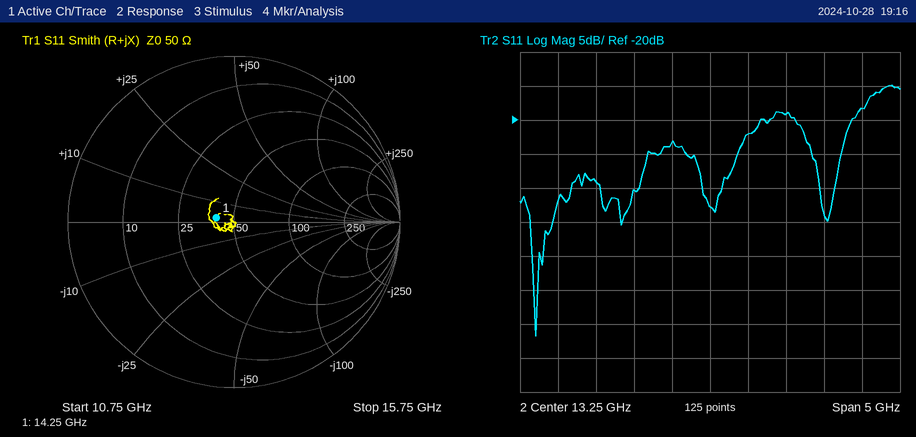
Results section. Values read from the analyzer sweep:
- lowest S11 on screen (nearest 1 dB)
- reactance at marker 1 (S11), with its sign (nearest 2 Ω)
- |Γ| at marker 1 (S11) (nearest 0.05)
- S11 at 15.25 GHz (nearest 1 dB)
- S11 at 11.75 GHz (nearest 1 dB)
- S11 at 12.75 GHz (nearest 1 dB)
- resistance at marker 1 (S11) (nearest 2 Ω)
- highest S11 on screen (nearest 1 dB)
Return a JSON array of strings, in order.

["-52 dB", "+2 Ω", "0.10", "-18 dB", "-29 dB", "-23 dB", "40 Ω", "-15 dB"]
